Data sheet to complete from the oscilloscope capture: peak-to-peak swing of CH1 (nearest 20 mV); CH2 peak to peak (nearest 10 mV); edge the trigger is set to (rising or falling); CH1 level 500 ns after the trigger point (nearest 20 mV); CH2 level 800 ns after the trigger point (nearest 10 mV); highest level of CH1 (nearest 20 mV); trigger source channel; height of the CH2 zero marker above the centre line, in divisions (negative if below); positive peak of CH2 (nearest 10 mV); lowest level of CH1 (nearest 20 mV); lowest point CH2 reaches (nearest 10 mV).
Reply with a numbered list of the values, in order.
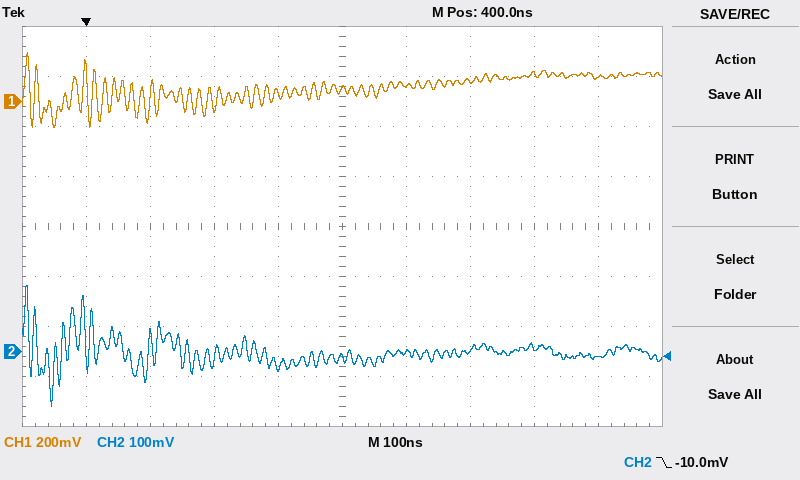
1. 300 mV
2. 240 mV
3. falling
4. 60 mV
5. -10 mV
6. 200 mV
7. CH2
8. -2.5 div
9. 130 mV
10. -100 mV
11. -110 mV
